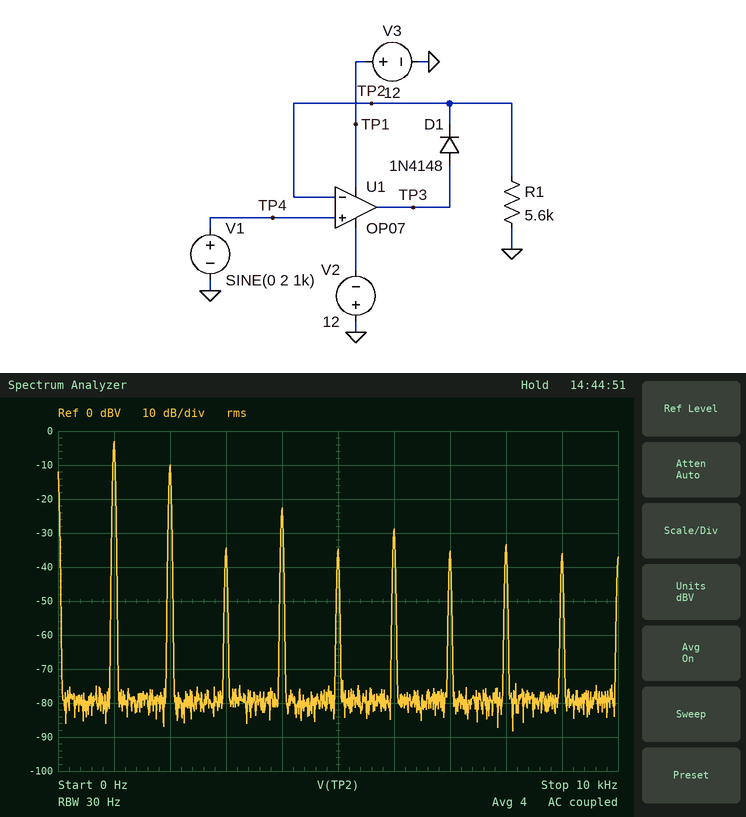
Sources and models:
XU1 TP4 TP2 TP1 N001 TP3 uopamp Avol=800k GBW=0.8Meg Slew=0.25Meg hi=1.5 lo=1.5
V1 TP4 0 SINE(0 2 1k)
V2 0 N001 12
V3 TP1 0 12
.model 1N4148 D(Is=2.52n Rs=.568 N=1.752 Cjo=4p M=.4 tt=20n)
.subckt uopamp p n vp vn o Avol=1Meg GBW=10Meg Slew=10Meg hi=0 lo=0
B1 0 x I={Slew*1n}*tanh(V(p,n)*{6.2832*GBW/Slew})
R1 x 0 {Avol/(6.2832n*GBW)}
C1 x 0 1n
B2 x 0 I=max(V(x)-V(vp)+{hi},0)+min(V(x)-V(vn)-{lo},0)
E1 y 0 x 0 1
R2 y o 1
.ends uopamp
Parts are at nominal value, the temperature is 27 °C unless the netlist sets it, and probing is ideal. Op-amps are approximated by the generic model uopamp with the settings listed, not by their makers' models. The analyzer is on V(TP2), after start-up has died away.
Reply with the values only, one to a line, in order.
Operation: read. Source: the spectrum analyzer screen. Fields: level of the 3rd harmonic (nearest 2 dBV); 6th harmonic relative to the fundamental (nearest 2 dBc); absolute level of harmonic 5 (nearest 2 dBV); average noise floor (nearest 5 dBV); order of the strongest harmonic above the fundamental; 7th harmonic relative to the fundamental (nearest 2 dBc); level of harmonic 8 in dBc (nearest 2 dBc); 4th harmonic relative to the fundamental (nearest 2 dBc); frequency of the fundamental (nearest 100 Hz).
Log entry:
-34 dBV
-26 dBc
-34 dBV
-80 dBV
2
-32 dBc
-30 dBc
-20 dBc
1.0 kHz
